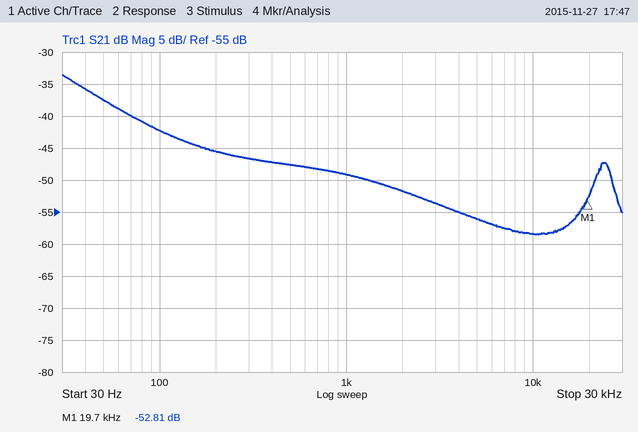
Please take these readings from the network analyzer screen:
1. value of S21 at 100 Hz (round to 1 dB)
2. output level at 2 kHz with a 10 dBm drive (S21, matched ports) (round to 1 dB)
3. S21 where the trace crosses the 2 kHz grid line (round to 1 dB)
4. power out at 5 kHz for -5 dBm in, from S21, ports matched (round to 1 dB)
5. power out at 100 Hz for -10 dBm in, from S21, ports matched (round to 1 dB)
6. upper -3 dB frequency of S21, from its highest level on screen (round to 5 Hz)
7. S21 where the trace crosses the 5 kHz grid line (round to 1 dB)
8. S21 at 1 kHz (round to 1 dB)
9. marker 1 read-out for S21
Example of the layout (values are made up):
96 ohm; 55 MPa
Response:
-42 dB; -42 dBm; -52 dB; -61 dBm; -52 dBm; 45 Hz; -56 dB; -49 dB; -52.81 dB
